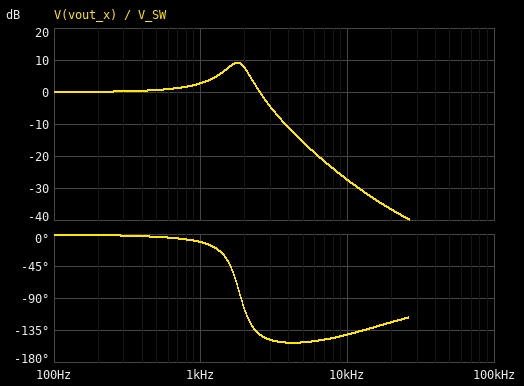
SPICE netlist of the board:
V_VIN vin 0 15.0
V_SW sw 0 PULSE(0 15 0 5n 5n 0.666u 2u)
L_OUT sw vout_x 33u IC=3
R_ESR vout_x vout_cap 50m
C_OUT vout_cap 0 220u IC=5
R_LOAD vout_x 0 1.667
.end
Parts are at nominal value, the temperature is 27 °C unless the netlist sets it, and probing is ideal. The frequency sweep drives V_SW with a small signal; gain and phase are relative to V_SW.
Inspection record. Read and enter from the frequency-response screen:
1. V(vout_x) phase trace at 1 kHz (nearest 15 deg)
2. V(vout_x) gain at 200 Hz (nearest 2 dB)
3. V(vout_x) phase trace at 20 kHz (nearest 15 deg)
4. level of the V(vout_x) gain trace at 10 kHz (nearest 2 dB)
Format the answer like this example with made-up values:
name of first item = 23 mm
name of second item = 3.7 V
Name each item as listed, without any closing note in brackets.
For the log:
V(vout_x) phase trace at 1 kHz = -15 deg
V(vout_x) gain at 200 Hz = 0 dB
V(vout_x) phase trace at 20 kHz = -120 deg
level of the V(vout_x) gain trace at 10 kHz = -28 dB
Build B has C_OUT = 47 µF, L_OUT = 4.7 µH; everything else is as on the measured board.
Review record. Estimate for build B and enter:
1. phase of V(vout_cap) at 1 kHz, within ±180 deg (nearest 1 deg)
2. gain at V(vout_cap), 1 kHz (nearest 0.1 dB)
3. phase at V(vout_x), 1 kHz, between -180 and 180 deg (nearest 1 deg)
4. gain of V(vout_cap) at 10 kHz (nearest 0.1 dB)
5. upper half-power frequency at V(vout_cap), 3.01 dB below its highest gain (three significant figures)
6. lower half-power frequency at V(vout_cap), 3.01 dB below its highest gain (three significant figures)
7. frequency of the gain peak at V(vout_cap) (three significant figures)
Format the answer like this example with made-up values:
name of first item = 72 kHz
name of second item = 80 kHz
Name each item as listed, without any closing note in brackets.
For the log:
phase of V(vout_cap) at 1 kHz, within ±180 deg = -2 deg
gain at V(vout_cap), 1 kHz = 0.1 dB
phase at V(vout_x), 1 kHz, between -180 and 180 deg = -1 deg
gain of V(vout_cap) at 10 kHz = 9.4 dB
upper half-power frequency at V(vout_cap), 3.01 dB below its highest gain = 11.9 kHz
lower half-power frequency at V(vout_cap), 3.01 dB below its highest gain = 8.20 kHz
frequency of the gain peak at V(vout_cap) = 10.2 kHz
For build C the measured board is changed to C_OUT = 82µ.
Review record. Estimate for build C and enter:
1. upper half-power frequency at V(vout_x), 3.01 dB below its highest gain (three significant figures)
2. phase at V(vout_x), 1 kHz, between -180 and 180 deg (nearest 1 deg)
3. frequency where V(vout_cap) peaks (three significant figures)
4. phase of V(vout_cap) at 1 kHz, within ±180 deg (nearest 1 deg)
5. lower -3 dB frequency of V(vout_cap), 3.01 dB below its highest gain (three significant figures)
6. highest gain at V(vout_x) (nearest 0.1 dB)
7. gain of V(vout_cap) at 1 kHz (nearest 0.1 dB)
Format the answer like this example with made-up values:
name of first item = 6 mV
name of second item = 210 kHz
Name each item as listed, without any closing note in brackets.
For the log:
upper half-power frequency at V(vout_x), 3.01 dB below its highest gain = 3.49 kHz
phase at V(vout_x), 1 kHz, between -180 and 180 deg = -8 deg
frequency where V(vout_cap) peaks = 2.86 kHz
phase of V(vout_cap) at 1 kHz, within ±180 deg = -10 deg
lower -3 dB frequency of V(vout_cap), 3.01 dB below its highest gain = 2.04 kHz
highest gain at V(vout_x) = 7.1 dB
gain of V(vout_cap) at 1 kHz = 0.9 dB
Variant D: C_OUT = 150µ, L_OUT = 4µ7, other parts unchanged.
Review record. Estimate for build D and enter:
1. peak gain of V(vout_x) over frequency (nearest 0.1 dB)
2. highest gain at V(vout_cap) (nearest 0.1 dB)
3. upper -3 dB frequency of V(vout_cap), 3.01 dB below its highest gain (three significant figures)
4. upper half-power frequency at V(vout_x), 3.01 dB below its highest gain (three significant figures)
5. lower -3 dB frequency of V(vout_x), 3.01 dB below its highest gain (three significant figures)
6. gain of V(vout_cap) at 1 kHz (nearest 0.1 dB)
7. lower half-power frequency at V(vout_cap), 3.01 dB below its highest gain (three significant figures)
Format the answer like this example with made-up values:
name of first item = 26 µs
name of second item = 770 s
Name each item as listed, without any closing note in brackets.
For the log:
peak gain of V(vout_x) over frequency = 8.8 dB
highest gain at V(vout_cap) = 8.5 dB
upper -3 dB frequency of V(vout_cap), 3.01 dB below its highest gain = 6.74 kHz
upper half-power frequency at V(vout_x), 3.01 dB below its highest gain = 6.77 kHz
lower -3 dB frequency of V(vout_x), 3.01 dB below its highest gain = 4.42 kHz
gain of V(vout_cap) at 1 kHz = 0.2 dB
lower half-power frequency at V(vout_cap), 3.01 dB below its highest gain = 4.38 kHz
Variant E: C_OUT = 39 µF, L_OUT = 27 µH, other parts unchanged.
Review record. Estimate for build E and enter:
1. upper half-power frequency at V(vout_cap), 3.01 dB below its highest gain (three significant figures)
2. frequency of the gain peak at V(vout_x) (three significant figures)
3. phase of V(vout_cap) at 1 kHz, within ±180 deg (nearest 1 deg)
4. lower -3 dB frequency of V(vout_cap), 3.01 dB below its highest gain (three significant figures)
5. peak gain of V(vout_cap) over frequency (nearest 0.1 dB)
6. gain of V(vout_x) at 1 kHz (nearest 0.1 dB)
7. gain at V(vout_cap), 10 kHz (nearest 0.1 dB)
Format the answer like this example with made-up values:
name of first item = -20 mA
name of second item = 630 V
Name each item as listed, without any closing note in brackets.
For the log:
upper half-power frequency at V(vout_cap), 3.01 dB below its highest gain = 5.67 kHz
frequency of the gain peak at V(vout_x) = 4.45 kHz
phase of V(vout_cap) at 1 kHz, within ±180 deg = -7 deg
lower -3 dB frequency of V(vout_cap), 3.01 dB below its highest gain = 2.73 kHz
peak gain of V(vout_cap) over frequency = 5.5 dB
gain of V(vout_x) at 1 kHz = 0.3 dB
gain at V(vout_cap), 10 kHz = -10.8 dB
